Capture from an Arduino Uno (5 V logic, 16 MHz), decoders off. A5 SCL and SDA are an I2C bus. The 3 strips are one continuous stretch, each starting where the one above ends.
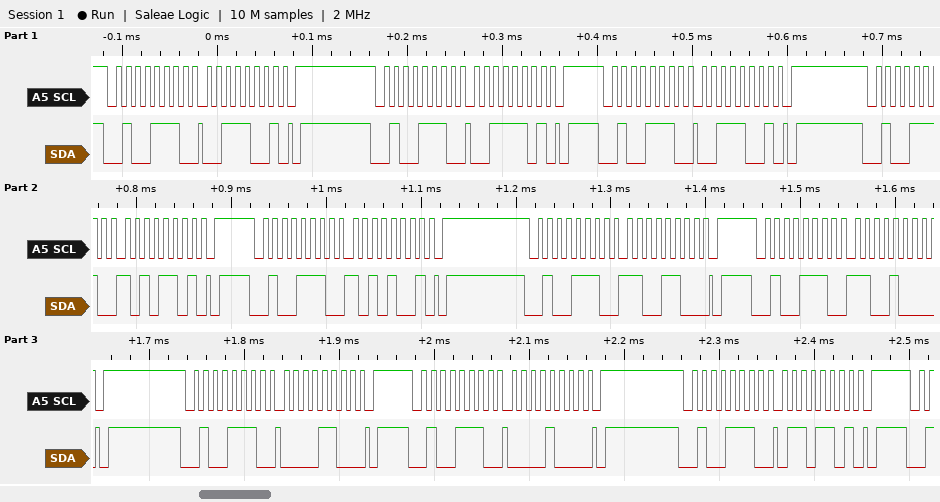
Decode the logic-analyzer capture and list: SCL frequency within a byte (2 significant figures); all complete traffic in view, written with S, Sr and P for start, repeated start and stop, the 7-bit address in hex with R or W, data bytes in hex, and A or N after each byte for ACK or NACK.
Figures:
100 kHz
S 27W A 39 A P S 27W A 3D A P S 27W A 39 A P S 27W A AD A P S 27W A A9 A P S 27W A CC A P S 27W A C8 A P S 27W A 0C A P S 27W A 08 A P S 27W A 6D A P
